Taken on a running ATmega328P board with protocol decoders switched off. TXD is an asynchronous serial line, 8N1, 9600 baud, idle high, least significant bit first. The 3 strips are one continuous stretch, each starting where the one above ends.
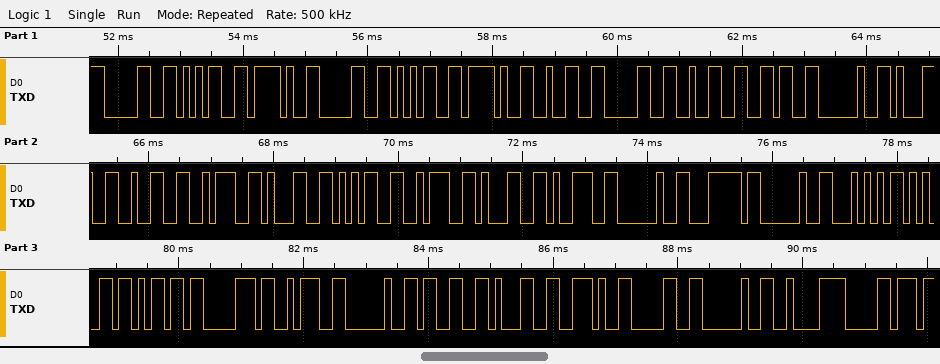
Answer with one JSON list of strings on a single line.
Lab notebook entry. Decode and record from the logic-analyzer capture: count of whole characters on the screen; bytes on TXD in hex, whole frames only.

["35", "30 35 2F 30 35 2F 32 30 32 36 20 31 32 3A 31 35 3A 31 39 20 7C 20 54 65 6D 70 3A 20 33 31 2E 30 20 C2 B0"]
